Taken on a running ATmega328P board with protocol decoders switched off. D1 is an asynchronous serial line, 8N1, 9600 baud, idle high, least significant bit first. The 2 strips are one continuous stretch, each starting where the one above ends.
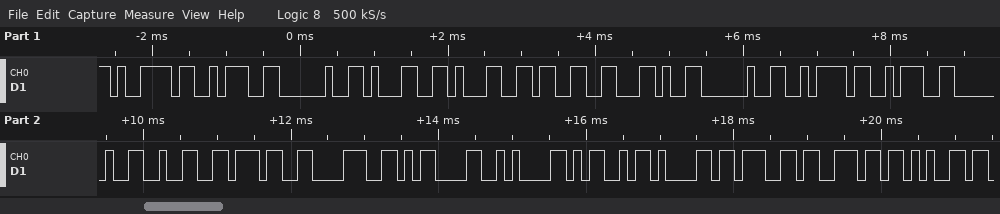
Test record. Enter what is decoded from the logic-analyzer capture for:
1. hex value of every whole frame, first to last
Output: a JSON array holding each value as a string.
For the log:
["79 3A 20 31 31 33 2C 20 7A 3A 20 32 37 38 0D 0A 4D 61 67 6E 65"]
